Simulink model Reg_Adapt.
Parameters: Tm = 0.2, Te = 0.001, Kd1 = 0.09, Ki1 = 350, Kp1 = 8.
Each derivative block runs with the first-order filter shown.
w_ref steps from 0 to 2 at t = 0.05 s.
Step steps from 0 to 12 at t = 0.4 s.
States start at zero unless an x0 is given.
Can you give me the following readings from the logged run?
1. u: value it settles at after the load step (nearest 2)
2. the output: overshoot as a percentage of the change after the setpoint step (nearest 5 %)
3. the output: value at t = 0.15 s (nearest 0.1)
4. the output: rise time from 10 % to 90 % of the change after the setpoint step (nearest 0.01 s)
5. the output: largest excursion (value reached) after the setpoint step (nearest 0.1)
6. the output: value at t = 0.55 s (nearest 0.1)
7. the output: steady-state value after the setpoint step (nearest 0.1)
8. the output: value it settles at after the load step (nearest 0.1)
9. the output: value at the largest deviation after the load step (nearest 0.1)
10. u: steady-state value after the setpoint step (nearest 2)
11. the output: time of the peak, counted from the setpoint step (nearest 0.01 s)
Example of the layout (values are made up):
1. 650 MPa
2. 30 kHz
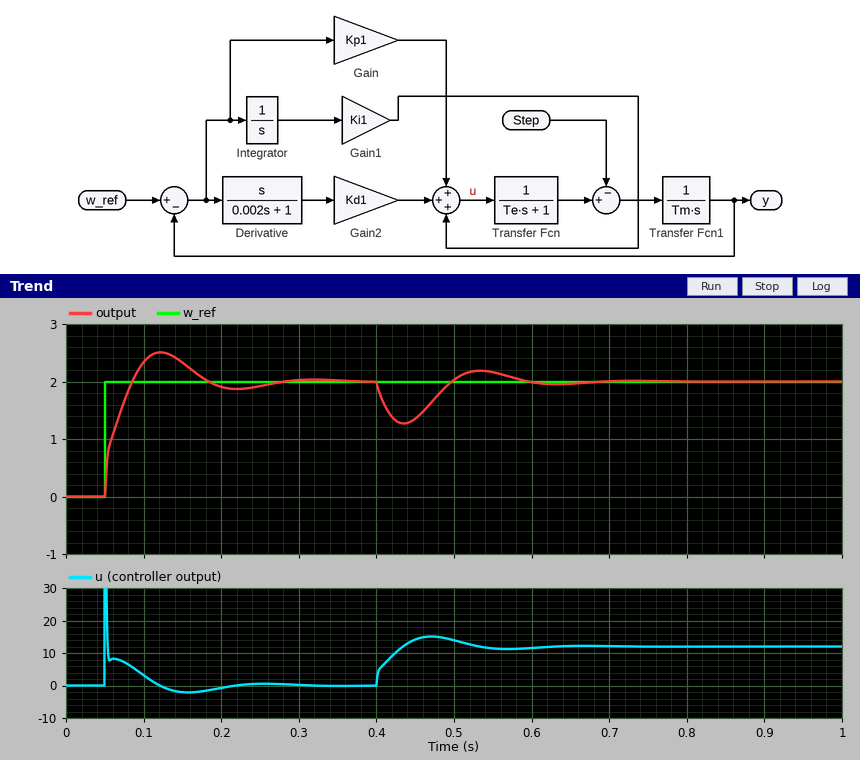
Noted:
1. 12
2. 25 %
3. 2.3
4. 0.03 s
5. 2.5
6. 2.2
7. 2.0
8. 2.0
9. 1.3
10. 0
11. 0.07 s
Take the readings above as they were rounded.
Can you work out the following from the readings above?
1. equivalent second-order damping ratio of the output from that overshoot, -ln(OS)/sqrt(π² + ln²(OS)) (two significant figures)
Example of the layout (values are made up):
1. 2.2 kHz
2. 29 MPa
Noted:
1. 0.40
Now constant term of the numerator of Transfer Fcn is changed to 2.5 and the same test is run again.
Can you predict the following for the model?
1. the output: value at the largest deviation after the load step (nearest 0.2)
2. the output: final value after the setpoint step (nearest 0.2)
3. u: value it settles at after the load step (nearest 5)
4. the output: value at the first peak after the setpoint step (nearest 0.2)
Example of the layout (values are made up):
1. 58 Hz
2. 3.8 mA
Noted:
1. 1.6
2. 2.0
3. 5
4. 2.2
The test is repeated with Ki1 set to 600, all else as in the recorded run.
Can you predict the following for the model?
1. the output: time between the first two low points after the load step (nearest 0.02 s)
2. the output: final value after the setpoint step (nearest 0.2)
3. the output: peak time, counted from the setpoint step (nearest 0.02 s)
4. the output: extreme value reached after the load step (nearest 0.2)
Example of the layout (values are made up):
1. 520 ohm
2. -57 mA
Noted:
1. 0.14 s
2. 2.0
3. 0.06 s
4. 1.4
